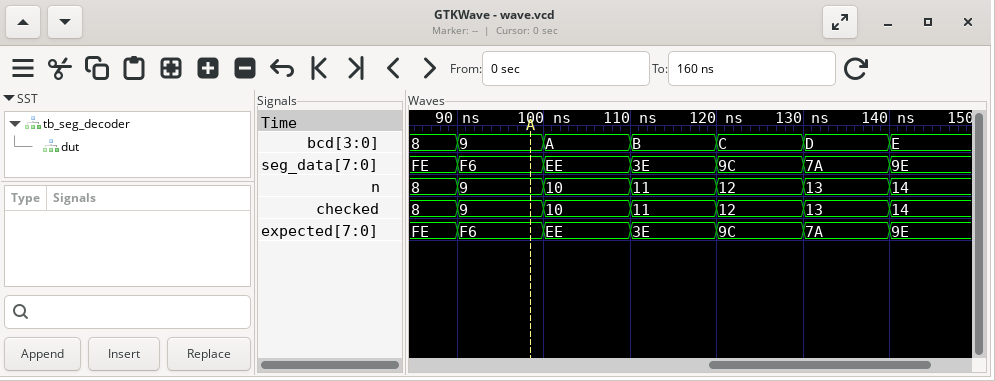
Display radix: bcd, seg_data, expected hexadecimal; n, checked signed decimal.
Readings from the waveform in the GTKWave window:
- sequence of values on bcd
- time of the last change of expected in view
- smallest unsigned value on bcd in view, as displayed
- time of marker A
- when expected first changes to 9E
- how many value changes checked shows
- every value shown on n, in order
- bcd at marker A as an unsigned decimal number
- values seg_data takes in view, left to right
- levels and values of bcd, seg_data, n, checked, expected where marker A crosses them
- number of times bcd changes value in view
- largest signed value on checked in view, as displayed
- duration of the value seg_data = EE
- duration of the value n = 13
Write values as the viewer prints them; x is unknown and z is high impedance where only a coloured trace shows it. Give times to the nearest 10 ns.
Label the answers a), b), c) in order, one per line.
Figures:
a) 8, 9, A, B, C, D, E
b) 140 ns
c) 8
d) 100 ns
e) 140 ns
f) 6
g) 8, 9, 10, 11, 12, 13, 14
h) 9
i) FE, F6, EE, 3E, 9C, 7A, 9E
j) bcd=9, seg_data=F6, n=9, checked=9, expected=F6
k) 6
l) 14
m) 10 ns
n) 10 ns
